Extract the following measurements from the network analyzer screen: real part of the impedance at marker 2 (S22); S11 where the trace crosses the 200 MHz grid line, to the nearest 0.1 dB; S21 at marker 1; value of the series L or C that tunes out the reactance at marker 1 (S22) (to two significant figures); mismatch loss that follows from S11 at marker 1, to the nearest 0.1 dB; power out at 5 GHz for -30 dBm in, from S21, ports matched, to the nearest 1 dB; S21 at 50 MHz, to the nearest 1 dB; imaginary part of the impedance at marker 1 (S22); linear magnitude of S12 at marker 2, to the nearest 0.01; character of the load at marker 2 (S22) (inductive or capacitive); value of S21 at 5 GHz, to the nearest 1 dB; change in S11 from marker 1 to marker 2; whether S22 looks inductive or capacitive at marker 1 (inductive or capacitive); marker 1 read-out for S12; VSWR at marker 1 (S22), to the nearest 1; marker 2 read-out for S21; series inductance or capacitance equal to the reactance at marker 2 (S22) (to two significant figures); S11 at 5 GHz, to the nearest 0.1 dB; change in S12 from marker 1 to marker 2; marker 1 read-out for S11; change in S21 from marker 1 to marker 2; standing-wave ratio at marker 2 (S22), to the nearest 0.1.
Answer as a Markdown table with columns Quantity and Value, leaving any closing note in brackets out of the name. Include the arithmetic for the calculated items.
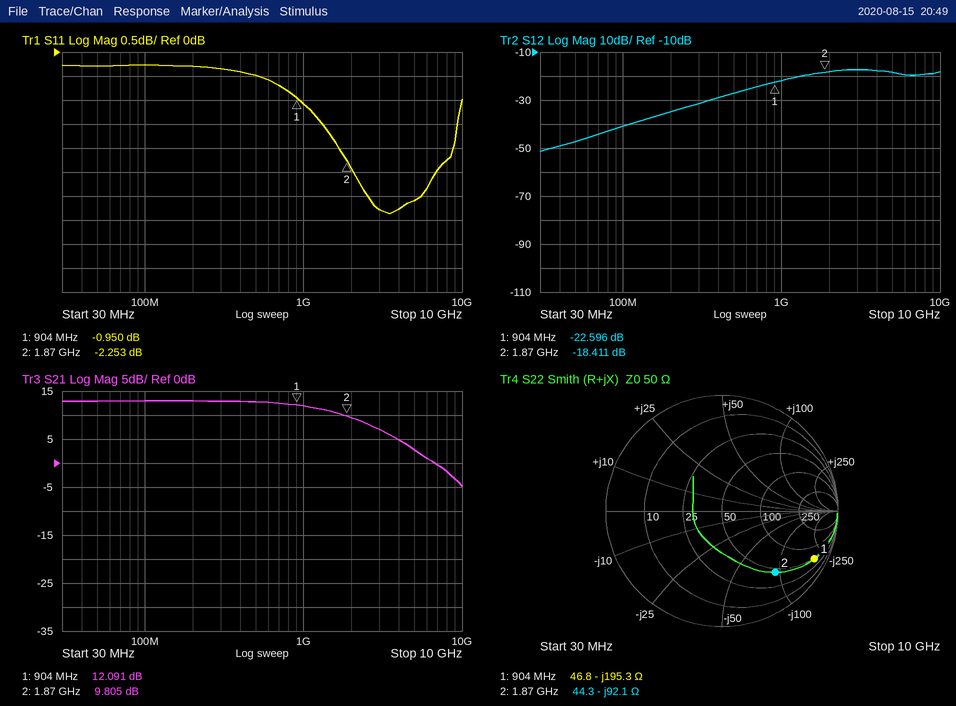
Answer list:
| Quantity | Value |
|---|---|
| real part of the impedance at marker 2 | 44.3 Ω |
| S11 where the trace crosses the 200 MHz grid line, to the nearest 0.1 dB | -0.3 dB |
| S21 at marker 1 | 12.091 dB |
| value of the series L or C that tunes out the reactance at marker 1 (S22) | L = 195.3 Ω/(2π × 904 MHz) ≈ 34 nH |
| mismatch loss that follows from S11 at marker 1, to the nearest 0.1 dB | −10 log10(1 − 10^(-0.95/10)) ≈ 7.1 dB |
| power out at 5 GHz for -30 dBm in, from S21, ports matched, to the nearest 1 dB | -30 dBm + (3 dB) = -27 dBm |
| S21 at 50 MHz, to the nearest 1 dB | 13 dB |
| imaginary part of the impedance at marker 1 | -195.3 Ω |
| linear magnitude of S12 at marker 2, to the nearest 0.01 | 10^(-18.411/20) ≈ 0.12 |
| character of the load at marker 2 (S22) | capacitive |
| value of S21 at 5 GHz, to the nearest 1 dB | 3 dB |
| change in S11 from marker 1 to marker 2 | -2.253 − (-0.95) = -1.303 dB |
| whether S22 looks inductive or capacitive at marker 1 | capacitive |
| marker 1 read-out for S12 | -22.596 dB |
| VSWR at marker 1 (S22), to the nearest 1 | 18 |
| marker 2 read-out for S21 | 9.805 dB |
| series inductance or capacitance equal to the reactance at marker 2 (S22) | C = 1/(2π × 1.87 GHz × 92.1 Ω) ≈ 924 fF, so 920 fF to two significant figures |
| S11 at 5 GHz, to the nearest 0.1 dB | -3.1 dB |
| change in S12 from marker 1 to marker 2 | -18.411 − (-22.596) = 4.185 dB |
| marker 1 read-out for S11 | -0.950 dB |
| change in S21 from marker 1 to marker 2 | 9.805 − (12.091) = -2.286 dB |
| standing-wave ratio at marker 2 (S22), to the nearest 0.1 | 5.7 |
